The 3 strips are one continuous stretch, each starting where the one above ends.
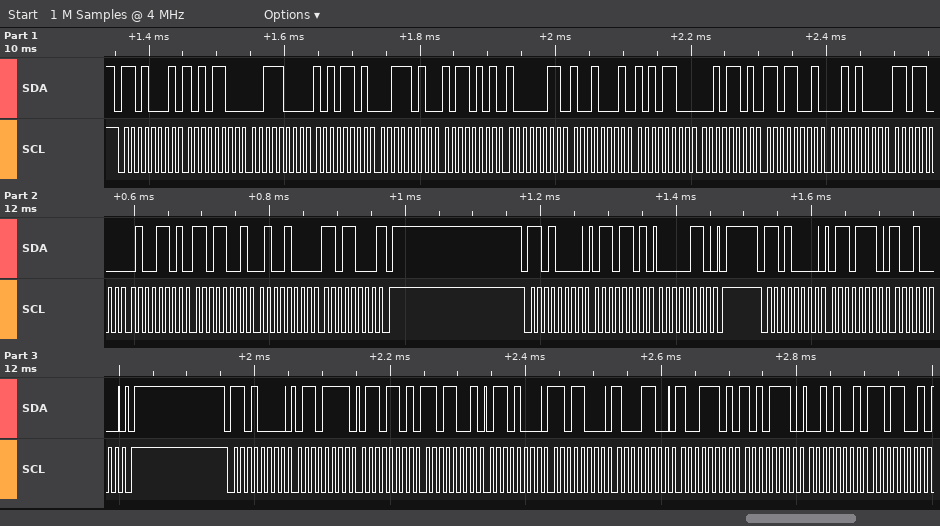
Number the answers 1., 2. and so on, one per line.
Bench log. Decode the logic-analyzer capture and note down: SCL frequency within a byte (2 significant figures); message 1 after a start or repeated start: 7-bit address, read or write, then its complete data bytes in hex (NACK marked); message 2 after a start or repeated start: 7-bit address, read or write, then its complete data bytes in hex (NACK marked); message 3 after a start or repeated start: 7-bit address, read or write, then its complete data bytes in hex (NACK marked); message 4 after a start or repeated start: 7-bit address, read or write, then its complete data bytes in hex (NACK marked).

1. 100 kHz
2. 0x68 read: AC 38 AD 3A B5 83 91 AC 2D D9 28 D8 4D D9 48 D8 NACK
3. 0x68 write: 6D 06
4. 0x68 write: 6E 90
5. 0x68 write: 6F 6D D9 68 D8 8C 9D AE 29 D9
